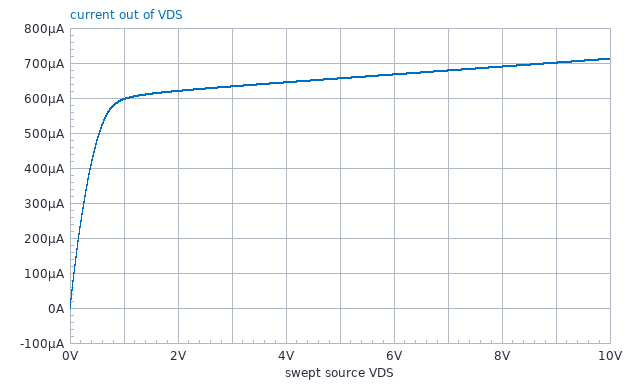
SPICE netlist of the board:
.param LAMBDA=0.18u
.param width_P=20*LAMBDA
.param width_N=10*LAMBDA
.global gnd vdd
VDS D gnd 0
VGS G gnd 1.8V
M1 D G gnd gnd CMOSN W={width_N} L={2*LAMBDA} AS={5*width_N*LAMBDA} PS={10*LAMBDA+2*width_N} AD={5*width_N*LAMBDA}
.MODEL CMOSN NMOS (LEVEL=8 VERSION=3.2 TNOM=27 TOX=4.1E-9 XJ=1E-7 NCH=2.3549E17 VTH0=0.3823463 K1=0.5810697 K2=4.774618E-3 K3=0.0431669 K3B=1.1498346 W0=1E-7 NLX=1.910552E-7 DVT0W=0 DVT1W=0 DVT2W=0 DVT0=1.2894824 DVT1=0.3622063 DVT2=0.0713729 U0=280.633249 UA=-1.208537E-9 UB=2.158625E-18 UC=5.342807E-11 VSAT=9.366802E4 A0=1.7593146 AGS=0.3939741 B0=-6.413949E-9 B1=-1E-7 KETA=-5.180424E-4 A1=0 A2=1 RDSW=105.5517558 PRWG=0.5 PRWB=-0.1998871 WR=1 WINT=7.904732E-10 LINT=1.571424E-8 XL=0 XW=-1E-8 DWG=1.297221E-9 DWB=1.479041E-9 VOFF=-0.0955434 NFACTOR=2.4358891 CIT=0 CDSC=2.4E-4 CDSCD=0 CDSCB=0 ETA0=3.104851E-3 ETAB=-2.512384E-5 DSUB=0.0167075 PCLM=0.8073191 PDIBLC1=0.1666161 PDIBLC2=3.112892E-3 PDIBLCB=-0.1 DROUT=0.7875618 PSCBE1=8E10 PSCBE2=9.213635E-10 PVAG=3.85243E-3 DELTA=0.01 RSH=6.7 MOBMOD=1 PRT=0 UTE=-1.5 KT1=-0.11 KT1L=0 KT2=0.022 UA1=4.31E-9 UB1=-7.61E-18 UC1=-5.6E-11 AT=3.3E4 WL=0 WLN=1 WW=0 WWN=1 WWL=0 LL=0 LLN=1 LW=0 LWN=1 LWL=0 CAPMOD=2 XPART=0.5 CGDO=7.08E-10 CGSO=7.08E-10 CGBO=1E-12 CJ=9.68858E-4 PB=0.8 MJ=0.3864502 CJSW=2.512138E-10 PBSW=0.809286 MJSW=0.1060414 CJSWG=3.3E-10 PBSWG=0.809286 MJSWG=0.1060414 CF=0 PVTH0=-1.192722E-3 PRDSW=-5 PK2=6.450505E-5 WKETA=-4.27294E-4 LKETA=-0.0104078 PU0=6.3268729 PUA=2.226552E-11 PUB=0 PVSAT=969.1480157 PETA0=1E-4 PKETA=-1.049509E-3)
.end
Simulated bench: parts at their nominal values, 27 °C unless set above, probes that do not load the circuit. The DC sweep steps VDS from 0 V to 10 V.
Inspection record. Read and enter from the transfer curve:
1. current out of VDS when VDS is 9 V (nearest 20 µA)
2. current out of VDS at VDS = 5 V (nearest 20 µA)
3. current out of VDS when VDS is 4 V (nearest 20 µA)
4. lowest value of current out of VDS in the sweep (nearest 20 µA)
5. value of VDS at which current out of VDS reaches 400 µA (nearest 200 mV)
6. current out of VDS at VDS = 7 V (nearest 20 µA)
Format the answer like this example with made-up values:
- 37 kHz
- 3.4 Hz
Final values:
- 700 µA
- 660 µA
- 640 µA
- 0 A
- 400 mV
- 680 µA
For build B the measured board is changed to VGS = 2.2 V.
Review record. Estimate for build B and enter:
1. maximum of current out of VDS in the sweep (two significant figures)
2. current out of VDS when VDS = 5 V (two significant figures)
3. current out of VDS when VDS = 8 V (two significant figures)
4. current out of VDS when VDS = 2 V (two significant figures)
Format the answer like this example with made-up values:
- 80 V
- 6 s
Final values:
- 970 µA
- 910 µA
- 950 µA
- 870 µA
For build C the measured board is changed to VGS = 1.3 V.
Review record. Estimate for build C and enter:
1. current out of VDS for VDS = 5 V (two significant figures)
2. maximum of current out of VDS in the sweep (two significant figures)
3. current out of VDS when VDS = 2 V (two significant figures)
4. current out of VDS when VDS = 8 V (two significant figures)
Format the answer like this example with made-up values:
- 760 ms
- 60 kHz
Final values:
- 340 µA
- 390 µA
- 310 µA
- 370 µA
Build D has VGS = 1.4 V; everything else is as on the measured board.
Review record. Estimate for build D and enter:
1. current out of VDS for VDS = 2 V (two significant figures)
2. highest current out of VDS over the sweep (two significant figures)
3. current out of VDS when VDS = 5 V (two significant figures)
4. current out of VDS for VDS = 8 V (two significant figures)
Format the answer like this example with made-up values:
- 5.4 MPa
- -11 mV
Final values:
- 370 µA
- 450 µA
- 400 µA
- 430 µA
